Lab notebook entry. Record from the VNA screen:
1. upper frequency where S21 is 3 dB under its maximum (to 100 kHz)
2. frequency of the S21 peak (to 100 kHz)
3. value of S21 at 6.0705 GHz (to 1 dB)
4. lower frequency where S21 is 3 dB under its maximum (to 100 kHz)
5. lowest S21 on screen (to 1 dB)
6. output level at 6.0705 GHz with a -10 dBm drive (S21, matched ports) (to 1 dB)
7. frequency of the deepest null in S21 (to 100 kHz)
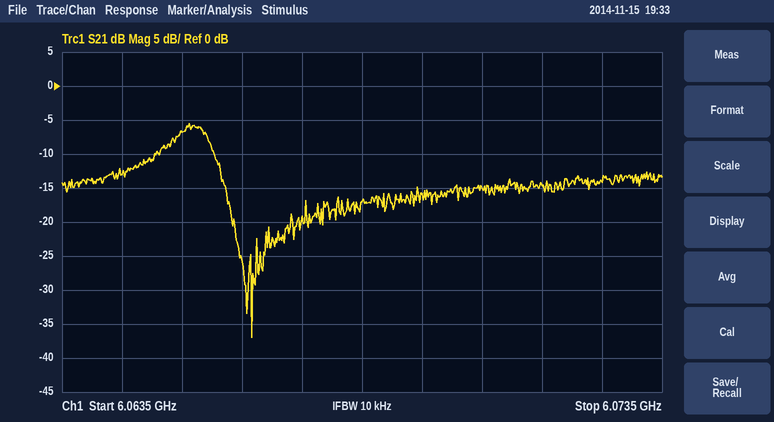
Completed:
6.0660 GHz
6.0656 GHz
-15 dB
6.0653 GHz
-37 dB
-25 dBm
6.0667 GHz
